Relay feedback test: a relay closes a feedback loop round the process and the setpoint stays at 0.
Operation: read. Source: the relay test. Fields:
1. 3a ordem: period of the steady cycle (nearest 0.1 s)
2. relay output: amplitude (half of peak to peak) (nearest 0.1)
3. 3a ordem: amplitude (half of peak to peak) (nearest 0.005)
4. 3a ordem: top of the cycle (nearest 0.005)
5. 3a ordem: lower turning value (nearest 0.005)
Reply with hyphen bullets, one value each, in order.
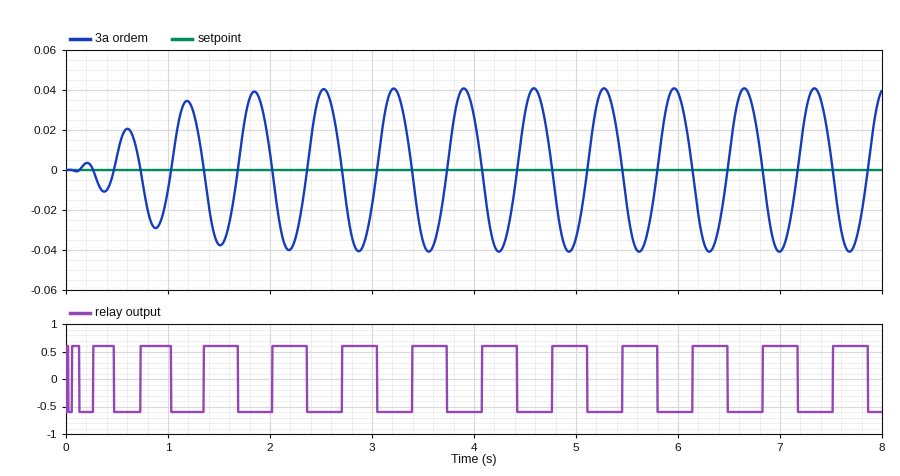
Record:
- 0.7 s
- 0.6
- 0.040
- 0.040
- -0.040
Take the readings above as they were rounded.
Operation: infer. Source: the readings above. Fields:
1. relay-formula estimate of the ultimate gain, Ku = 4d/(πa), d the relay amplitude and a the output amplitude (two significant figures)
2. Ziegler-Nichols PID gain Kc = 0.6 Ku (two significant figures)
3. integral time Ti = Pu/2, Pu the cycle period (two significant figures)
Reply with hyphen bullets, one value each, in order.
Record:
- 19
- 11
- 0.35 s
